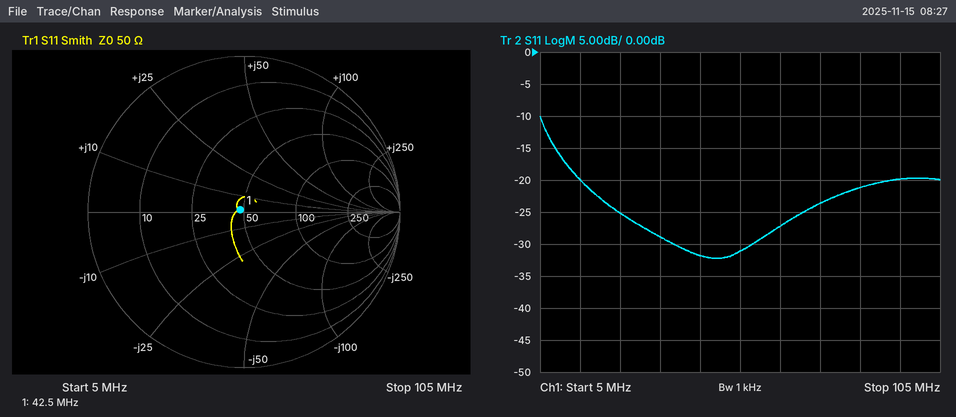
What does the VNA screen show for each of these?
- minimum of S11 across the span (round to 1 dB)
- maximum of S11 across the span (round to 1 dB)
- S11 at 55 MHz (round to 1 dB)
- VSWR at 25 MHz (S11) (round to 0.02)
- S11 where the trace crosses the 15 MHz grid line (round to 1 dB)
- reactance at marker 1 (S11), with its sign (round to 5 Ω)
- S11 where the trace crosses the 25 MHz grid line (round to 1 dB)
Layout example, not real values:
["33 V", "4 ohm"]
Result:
["-32 dB", "-10 dB", "-31 dB", "1.12", "-20 dB", "0 Ω", "-25 dB"]
